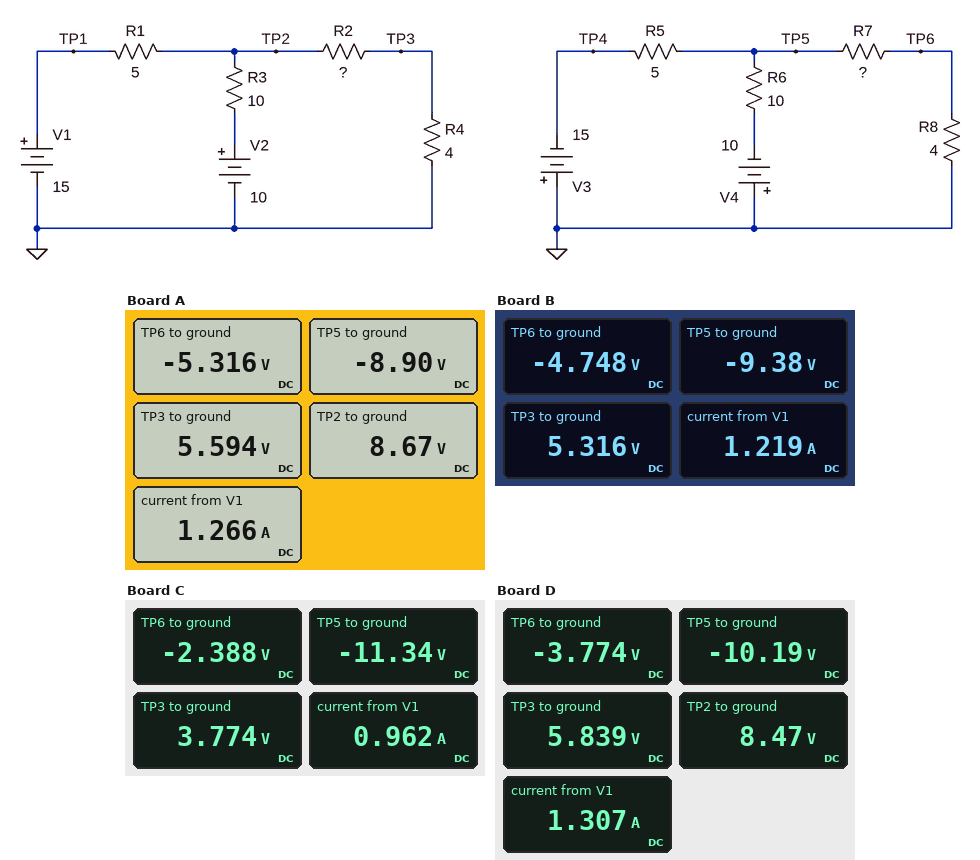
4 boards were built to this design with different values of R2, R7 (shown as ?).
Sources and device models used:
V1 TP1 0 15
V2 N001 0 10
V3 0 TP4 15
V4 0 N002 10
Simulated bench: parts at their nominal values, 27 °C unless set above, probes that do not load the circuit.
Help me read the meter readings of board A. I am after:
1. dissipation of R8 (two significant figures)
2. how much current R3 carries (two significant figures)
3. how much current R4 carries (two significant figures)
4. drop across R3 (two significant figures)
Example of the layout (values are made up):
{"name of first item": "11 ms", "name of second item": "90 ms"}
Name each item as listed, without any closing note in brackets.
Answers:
{"dissipation of R8": "7.1 W", "how much current R3 carries": "130 mA", "how much current R4 carries": "1.4 A", "drop across R3": "1.3 V"}
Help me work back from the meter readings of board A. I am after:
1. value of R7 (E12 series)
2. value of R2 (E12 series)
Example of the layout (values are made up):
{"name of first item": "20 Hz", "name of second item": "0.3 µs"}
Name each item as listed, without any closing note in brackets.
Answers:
{"value of R7": "2.7 Ω", "value of R2": "2.2 Ω"}
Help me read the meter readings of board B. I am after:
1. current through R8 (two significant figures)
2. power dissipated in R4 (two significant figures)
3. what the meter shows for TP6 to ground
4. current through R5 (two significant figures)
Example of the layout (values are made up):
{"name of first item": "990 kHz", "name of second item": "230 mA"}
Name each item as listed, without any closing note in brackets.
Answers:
{"current through R8": "1.2 A", "power dissipated in R4": "7.1 W", "what the meter shows for TP6 to ground": "-4.748 V", "current through R5": "1.1 A"}
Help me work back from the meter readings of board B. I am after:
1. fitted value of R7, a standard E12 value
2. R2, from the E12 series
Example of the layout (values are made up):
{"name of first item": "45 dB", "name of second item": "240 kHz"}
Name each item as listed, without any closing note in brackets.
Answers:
{"fitted value of R7, a standard E12 value": "3.9 Ω", "R2, from the E12 series": "2.7 Ω"}
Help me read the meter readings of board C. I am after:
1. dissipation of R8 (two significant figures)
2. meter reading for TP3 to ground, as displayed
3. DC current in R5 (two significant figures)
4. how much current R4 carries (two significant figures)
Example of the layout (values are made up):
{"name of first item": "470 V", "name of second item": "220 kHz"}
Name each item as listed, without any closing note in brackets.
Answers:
{"dissipation of R8": "1.4 W", "meter reading for TP3 to ground, as displayed": "3.774 V", "DC current in R5": "730 mA", "how much current R4 carries": "940 mA"}
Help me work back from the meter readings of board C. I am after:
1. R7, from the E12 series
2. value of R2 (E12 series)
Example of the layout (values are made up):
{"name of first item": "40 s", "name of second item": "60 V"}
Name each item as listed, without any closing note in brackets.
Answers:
{"R7, from the E12 series": "15 Ω", "value of R2": "6.8 Ω"}
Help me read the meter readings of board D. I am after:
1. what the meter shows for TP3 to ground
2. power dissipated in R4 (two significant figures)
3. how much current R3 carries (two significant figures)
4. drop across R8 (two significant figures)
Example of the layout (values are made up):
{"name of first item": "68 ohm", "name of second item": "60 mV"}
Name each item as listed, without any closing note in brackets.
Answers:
{"what the meter shows for TP3 to ground": "5.839 V", "power dissipated in R4": "8.5 W", "how much current R3 carries": "150 mA", "drop across R8": "3.8 V"}
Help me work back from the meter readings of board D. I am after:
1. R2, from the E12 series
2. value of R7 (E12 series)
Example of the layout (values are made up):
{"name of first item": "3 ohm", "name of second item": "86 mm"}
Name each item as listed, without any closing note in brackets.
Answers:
{"R2, from the E12 series": "1.8 Ω", "value of R7": "6.8 Ω"}
